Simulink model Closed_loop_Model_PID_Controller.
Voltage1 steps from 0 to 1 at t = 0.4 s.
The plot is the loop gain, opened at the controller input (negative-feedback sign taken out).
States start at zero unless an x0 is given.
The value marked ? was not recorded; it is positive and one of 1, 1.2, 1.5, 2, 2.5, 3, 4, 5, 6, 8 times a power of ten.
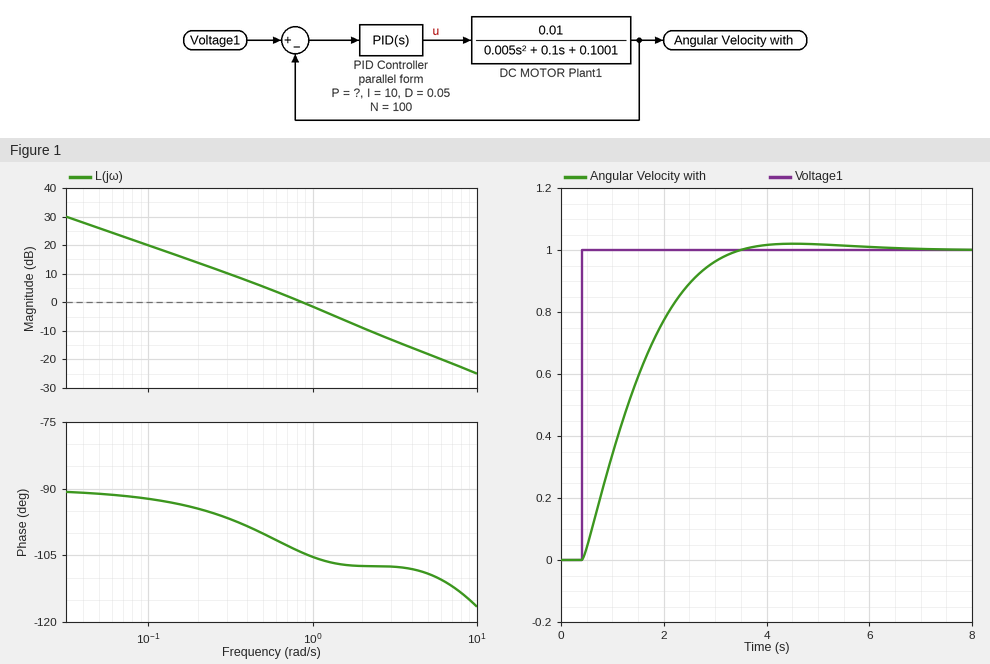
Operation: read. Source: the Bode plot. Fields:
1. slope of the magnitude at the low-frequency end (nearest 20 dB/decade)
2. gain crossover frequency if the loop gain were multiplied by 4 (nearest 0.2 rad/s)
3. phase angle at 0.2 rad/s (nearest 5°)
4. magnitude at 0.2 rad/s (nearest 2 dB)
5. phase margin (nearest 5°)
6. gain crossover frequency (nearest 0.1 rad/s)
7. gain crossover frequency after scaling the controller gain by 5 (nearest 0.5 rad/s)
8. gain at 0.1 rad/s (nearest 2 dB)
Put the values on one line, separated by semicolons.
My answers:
-20 dB/decade; 2.8 rad/s; -95°; 14 dB; 75°; 0.9 rad/s; 3.5 rad/s; 20 dB
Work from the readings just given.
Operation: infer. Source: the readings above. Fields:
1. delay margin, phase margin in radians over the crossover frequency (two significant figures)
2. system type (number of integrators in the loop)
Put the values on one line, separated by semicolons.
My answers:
1.5 s; 1
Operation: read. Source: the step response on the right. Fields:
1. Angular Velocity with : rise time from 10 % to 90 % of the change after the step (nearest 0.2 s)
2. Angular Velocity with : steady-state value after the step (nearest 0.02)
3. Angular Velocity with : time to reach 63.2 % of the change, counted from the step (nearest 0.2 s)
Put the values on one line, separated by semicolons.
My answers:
2.0 s; 1.00; 1.2 s
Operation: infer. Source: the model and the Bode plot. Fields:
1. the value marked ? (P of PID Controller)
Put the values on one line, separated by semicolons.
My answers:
6
